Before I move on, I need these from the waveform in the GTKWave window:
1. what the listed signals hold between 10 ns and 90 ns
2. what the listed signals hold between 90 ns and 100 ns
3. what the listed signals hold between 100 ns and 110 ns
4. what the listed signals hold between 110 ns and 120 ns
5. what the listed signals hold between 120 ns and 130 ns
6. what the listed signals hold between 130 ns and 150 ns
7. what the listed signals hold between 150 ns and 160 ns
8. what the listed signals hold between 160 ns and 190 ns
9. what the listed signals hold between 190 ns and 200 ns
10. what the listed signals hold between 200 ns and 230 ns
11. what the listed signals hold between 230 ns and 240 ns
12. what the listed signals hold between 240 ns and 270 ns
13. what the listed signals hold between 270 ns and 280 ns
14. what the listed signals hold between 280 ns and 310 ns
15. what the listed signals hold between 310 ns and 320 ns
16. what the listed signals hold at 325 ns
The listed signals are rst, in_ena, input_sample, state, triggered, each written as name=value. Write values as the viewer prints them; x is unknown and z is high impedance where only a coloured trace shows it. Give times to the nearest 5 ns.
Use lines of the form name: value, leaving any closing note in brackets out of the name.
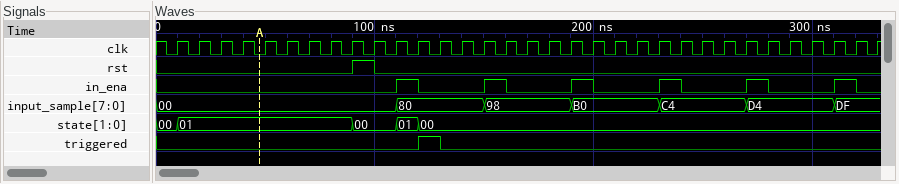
what the listed signals hold between 10 ns and 90 ns: rst=0, in_ena=0, input_sample=00, state=01, triggered=0
what the listed signals hold between 90 ns and 100 ns: rst=1, in_ena=0, input_sample=00, state=00, triggered=0
what the listed signals hold between 100 ns and 110 ns: rst=0, in_ena=0, input_sample=00, state=00, triggered=0
what the listed signals hold between 110 ns and 120 ns: rst=0, in_ena=1, input_sample=80, state=01, triggered=0
what the listed signals hold between 120 ns and 130 ns: rst=0, in_ena=0, input_sample=80, state=00, triggered=1
what the listed signals hold between 130 ns and 150 ns: rst=0, in_ena=0, input_sample=80, state=00, triggered=0
what the listed signals hold between 150 ns and 160 ns: rst=0, in_ena=1, input_sample=98, state=00, triggered=0
what the listed signals hold between 160 ns and 190 ns: rst=0, in_ena=0, input_sample=98, state=00, triggered=0
what the listed signals hold between 190 ns and 200 ns: rst=0, in_ena=1, input_sample=B0, state=00, triggered=0
what the listed signals hold between 200 ns and 230 ns: rst=0, in_ena=0, input_sample=B0, state=00, triggered=0
what the listed signals hold between 230 ns and 240 ns: rst=0, in_ena=1, input_sample=C4, state=00, triggered=0
what the listed signals hold between 240 ns and 270 ns: rst=0, in_ena=0, input_sample=C4, state=00, triggered=0
what the listed signals hold between 270 ns and 280 ns: rst=0, in_ena=1, input_sample=D4, state=00, triggered=0
what the listed signals hold between 280 ns and 310 ns: rst=0, in_ena=0, input_sample=D4, state=00, triggered=0
what the listed signals hold between 310 ns and 320 ns: rst=0, in_ena=1, input_sample=DF, state=00, triggered=0
what the listed signals hold at 325 ns: rst=0, in_ena=0, input_sample=DF, state=00, triggered=0
